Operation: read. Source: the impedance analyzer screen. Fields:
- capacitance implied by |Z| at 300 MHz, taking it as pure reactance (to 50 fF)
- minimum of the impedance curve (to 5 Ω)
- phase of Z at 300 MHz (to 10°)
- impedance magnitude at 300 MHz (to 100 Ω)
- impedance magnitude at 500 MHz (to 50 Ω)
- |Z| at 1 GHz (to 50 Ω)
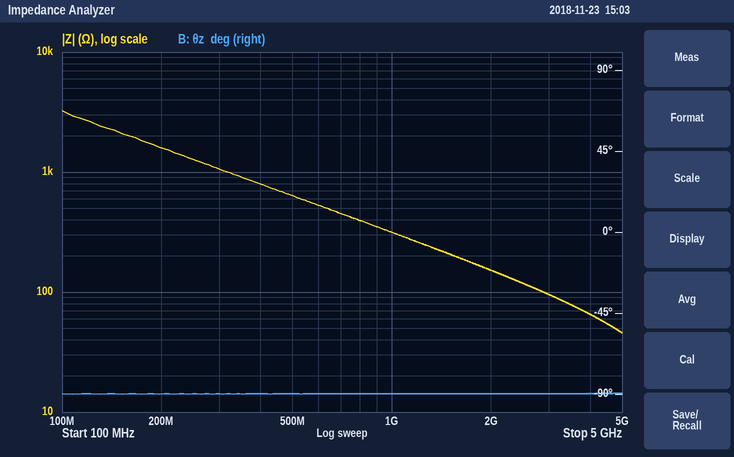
500 fF
45 Ω
-90°
1.1 kΩ
650 Ω
300 Ω
